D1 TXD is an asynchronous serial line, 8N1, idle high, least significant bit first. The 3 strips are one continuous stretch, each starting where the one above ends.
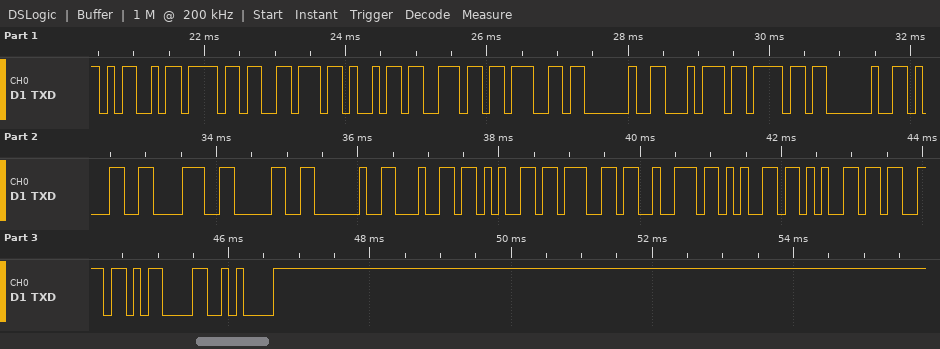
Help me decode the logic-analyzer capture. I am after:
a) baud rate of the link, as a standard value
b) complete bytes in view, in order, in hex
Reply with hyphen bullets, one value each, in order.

- 9600 baud
- 0x4D 0x6F 0x76 0x69 0x6E 0x67 0x20 0x74 0x6F 0x20 0x31 0x38 0x30 0x20 0x64 0x65 0x67 0x72 0x65 0x65 0x73 0x0D 0x0A
